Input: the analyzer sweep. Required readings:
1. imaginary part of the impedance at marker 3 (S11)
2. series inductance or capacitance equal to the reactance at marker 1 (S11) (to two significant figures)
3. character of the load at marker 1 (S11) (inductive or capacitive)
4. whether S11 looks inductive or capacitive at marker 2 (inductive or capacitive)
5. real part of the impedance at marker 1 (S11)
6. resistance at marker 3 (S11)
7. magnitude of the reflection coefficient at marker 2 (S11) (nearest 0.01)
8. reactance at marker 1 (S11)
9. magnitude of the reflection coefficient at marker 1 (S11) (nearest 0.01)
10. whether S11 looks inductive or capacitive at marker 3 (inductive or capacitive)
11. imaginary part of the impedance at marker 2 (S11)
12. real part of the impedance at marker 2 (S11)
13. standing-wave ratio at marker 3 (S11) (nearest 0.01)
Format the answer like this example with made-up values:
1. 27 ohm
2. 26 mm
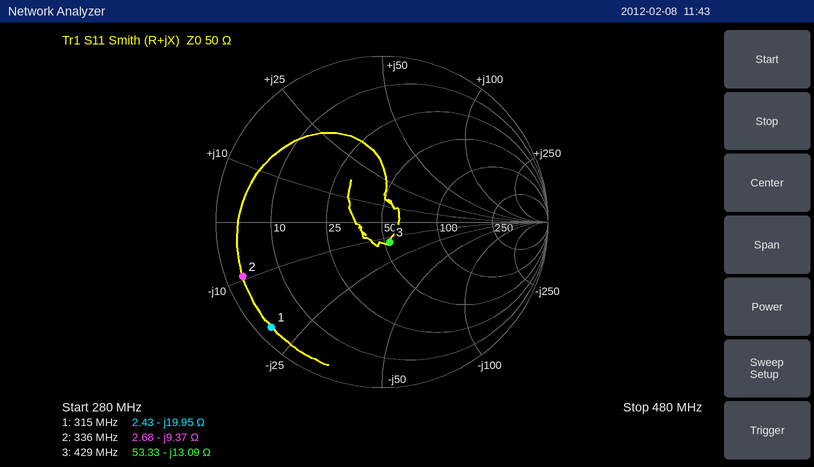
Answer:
1. -13.09 Ω
2. 25 pF
3. capacitive
4. capacitive
5. 2.43 Ω
6. 53.33 Ω
7. 0.90
8. -19.95 Ω
9. 0.92
10. capacitive
11. -9.37 Ω
12. 2.68 Ω
13. 1.30
